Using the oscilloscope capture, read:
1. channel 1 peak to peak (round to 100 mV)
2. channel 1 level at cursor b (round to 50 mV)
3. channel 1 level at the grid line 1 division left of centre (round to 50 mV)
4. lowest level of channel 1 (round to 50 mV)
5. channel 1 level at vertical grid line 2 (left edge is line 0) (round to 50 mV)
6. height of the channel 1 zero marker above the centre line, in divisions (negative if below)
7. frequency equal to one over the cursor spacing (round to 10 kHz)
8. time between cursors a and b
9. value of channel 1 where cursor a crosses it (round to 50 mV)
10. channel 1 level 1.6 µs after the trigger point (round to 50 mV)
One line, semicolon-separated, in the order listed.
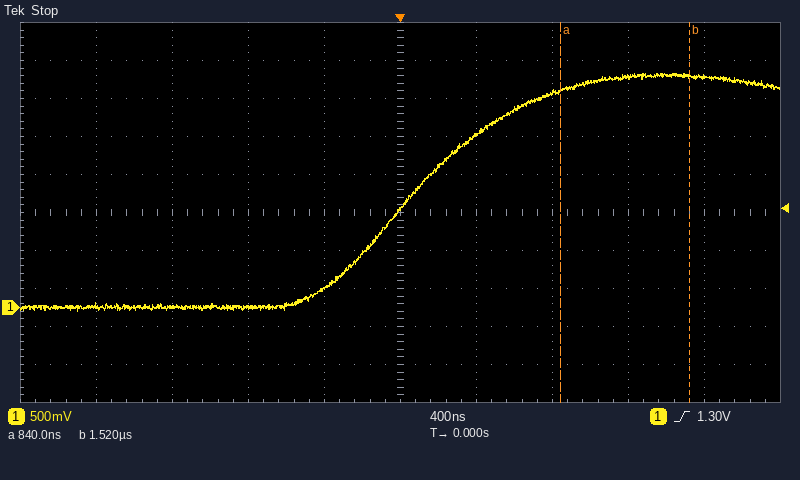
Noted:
3.10 V; 3.05 V; 250 mV; -50 mV; 0 mV; -2.5 div; 1.47 MHz; 680 ns; 2.85 V; 3.05 V
